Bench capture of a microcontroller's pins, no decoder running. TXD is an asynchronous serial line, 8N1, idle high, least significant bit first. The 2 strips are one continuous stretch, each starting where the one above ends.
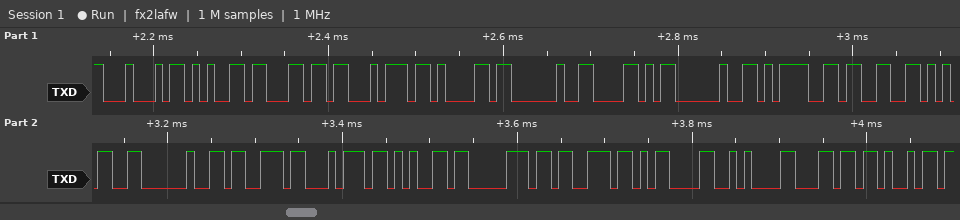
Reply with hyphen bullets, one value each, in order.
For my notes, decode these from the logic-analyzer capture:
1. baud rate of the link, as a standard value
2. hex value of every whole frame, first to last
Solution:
- 115200 baud
- 44 65 6C 74 61 20 58 20 3D 33 35 20 73 74 65 70 73 0D 0A 6C 69
